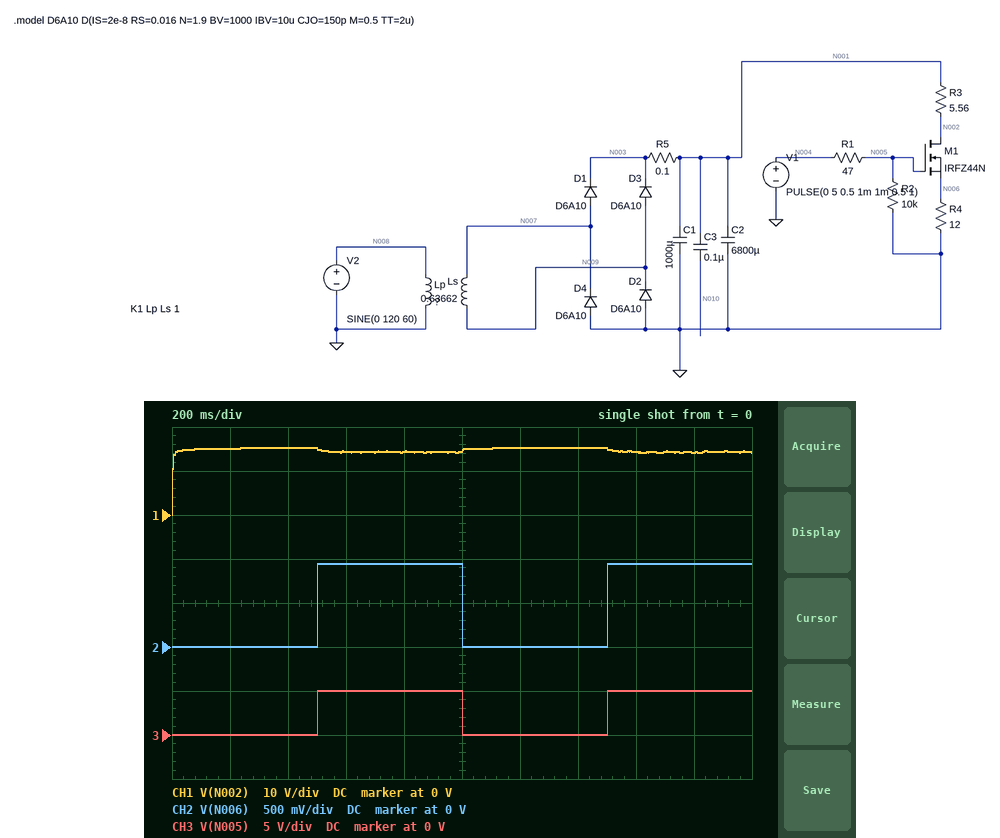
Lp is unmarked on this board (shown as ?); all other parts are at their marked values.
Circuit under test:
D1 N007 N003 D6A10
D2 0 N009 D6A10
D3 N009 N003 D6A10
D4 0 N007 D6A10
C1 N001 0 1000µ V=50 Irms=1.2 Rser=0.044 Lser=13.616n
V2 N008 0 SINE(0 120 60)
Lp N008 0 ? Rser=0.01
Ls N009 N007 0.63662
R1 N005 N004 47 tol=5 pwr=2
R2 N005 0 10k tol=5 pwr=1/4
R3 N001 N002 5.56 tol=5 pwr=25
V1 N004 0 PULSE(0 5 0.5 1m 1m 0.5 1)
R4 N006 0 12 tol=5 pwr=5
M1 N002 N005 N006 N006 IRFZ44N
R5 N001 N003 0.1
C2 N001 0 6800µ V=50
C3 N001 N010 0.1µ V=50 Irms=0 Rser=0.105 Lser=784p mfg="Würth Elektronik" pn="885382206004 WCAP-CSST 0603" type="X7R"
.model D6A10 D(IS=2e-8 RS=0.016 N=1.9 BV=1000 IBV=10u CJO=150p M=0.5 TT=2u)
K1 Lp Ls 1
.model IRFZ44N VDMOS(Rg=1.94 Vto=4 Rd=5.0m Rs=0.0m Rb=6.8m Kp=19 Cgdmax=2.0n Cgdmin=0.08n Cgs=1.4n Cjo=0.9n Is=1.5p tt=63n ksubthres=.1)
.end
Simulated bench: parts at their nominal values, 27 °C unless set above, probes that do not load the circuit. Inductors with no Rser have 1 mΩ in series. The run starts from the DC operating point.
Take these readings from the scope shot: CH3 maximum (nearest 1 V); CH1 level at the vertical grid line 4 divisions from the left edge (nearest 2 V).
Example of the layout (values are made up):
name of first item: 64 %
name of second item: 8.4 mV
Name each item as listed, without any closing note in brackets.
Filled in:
CH3 maximum: 5 V
CH1 level at the vertical grid line 4 divisions from the left edge: 14 V
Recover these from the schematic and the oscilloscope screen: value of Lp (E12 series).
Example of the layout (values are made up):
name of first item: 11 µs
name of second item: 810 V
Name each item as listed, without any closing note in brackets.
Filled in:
value of Lp: 33 H
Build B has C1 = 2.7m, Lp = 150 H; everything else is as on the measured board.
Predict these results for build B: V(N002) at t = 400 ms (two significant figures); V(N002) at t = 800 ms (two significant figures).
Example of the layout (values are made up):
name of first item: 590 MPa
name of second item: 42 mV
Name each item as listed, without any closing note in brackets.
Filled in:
V(N002) at t = 400 ms: 6.4 V
V(N002) at t = 800 ms: 5.6 V
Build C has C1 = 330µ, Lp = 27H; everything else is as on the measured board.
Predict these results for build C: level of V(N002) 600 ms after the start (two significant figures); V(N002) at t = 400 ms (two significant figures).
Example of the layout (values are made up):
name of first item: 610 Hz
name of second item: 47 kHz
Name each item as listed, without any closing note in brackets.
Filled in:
level of V(N002) 600 ms after the start: 16 V
V(N002) at t = 400 ms: 17 V
